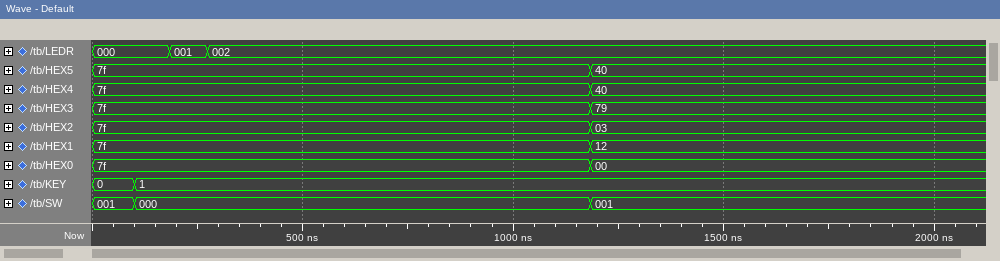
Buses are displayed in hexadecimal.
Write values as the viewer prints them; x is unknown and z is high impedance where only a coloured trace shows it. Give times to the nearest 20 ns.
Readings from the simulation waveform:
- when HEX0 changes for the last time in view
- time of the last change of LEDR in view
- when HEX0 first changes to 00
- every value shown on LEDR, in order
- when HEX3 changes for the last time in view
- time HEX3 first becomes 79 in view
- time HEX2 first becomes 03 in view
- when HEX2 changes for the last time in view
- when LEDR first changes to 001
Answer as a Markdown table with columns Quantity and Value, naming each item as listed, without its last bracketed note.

| Quantity | Value |
|---|---|
| when HEX0 changes for the last time in view | 1180 ns |
| time of the last change of LEDR in view | 280 ns |
| when HEX0 first changes to 00 | 1180 ns |
| every value shown on LEDR, in order | 000, 001, 002 |
| when HEX3 changes for the last time in view | 1180 ns |
| time HEX3 first becomes 79 in view | 1180 ns |
| time HEX2 first becomes 03 in view | 1180 ns |
| when HEX2 changes for the last time in view | 1180 ns |
| when LEDR first changes to 001 | 180 ns |
